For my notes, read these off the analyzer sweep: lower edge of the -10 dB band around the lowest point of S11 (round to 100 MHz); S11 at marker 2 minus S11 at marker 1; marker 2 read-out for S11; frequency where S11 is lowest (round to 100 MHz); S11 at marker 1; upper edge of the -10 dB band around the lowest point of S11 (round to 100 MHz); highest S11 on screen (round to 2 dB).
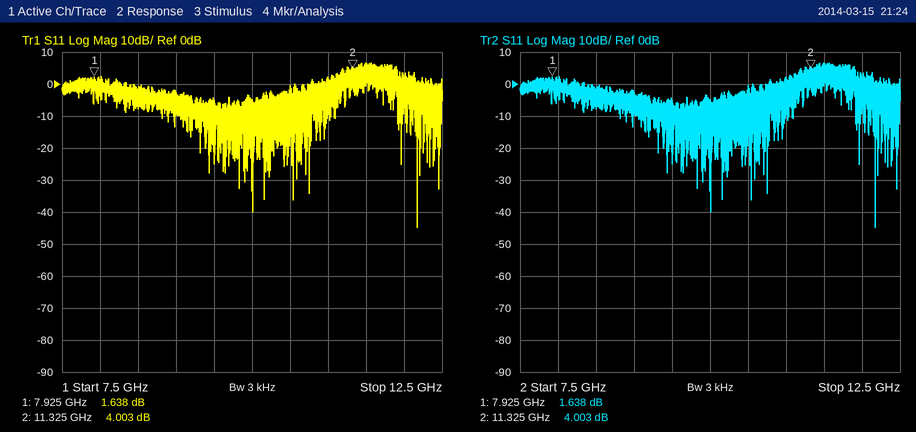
12.2 GHz
2.365 dB
4.003 dB
12.2 GHz
1.638 dB
12.2 GHz
6 dB
